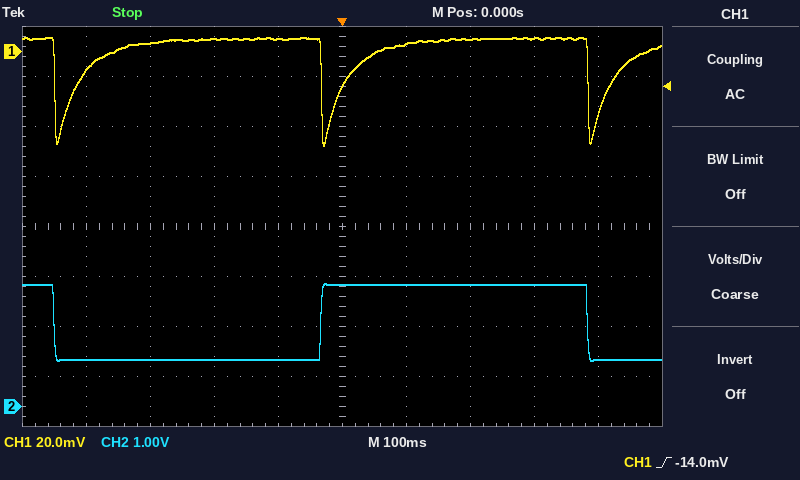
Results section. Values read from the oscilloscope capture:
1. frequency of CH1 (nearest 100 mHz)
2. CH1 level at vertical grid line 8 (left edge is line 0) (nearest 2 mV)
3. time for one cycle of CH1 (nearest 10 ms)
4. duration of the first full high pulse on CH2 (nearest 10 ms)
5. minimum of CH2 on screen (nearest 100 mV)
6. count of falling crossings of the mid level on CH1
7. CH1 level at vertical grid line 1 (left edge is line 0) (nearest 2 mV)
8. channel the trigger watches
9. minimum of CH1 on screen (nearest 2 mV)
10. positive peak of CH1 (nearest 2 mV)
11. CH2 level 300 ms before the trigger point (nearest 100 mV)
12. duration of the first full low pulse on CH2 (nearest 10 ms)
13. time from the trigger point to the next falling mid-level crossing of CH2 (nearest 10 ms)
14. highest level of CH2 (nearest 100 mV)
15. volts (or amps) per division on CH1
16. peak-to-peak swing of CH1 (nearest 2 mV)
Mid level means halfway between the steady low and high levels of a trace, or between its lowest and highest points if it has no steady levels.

2.4 Hz
6 mV
420 ms
420 ms
900 mV
3
-8 mV
CH1
-38 mV
6 mV
900 mV
420 ms
380 ms
2.5 V
20 mV
44 mV
